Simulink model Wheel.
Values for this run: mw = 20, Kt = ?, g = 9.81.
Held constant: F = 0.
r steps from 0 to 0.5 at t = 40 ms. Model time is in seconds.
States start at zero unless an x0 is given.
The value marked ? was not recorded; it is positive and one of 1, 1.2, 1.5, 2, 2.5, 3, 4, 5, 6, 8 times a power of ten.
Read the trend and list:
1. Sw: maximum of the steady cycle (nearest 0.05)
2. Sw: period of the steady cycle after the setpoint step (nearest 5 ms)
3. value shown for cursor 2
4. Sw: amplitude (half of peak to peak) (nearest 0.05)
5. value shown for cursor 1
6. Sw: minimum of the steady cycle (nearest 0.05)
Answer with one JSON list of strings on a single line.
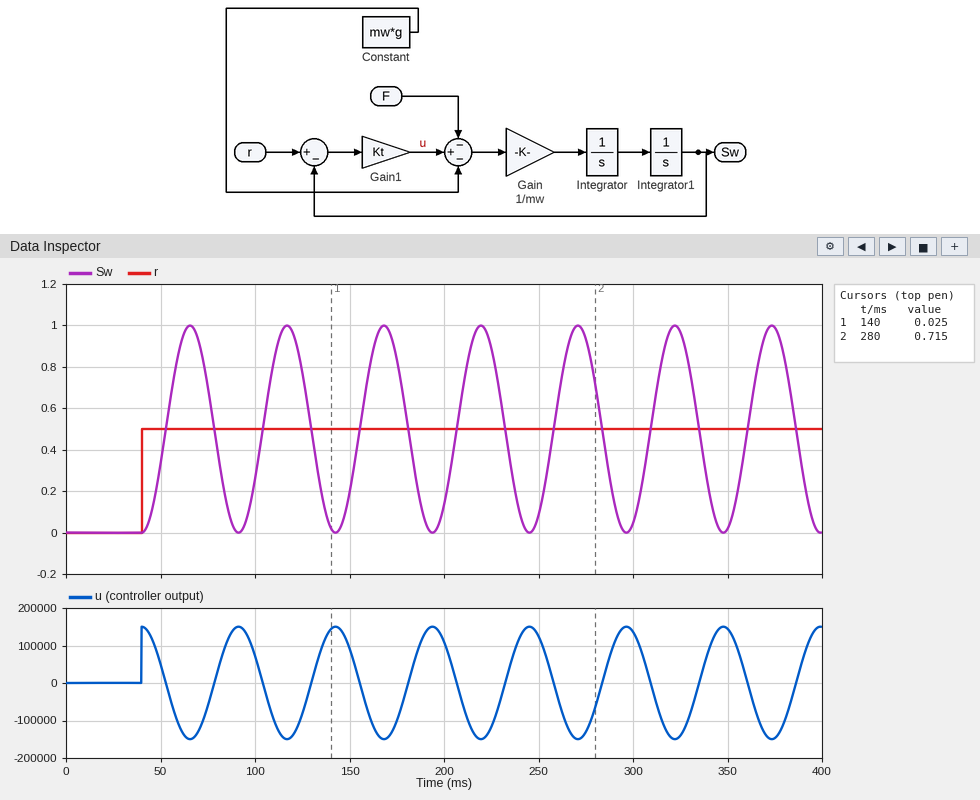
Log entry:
["1.00", "50 ms", "0.715", "0.50", "0.025", "0.00"]
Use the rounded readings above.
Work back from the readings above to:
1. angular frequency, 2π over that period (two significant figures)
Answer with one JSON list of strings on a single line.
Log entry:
["0.13 rad/ms"]
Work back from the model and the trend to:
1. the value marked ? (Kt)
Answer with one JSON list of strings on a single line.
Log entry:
["300000"]
